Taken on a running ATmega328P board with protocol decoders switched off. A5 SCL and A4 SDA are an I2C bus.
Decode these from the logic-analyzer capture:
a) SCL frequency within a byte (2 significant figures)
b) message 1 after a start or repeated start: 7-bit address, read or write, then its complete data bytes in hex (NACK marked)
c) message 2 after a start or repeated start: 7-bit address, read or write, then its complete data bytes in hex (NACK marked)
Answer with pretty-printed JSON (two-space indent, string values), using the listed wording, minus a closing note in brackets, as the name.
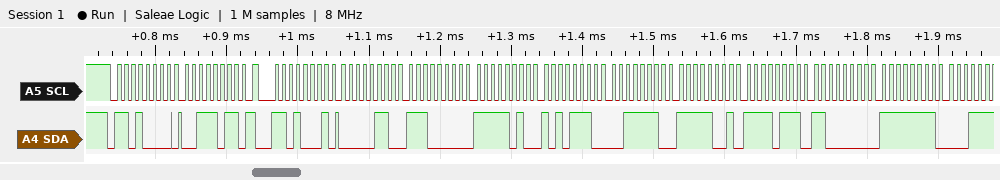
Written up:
{
  "SCL frequency within a byte": "100 kHz",
  "message 1 after a start or repeated start: 7-bit address, read or write, then its complete data bytes in hex": "0x68 write: 3B",
  "message 2 after a start or repeated start: 7-bit address, read or write, then its complete data bytes in hex": "0x68 read: 06 E0 FA AE 3E F9 F7 C0 FF"
}
